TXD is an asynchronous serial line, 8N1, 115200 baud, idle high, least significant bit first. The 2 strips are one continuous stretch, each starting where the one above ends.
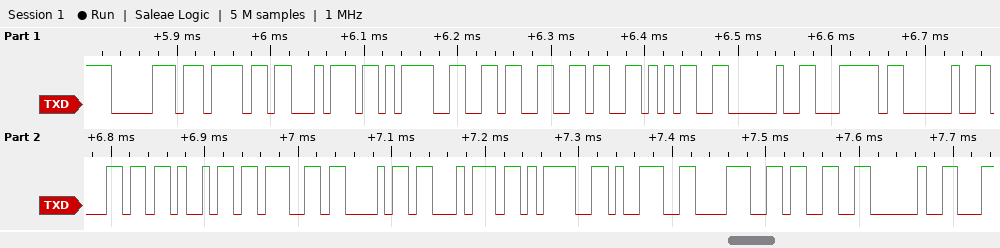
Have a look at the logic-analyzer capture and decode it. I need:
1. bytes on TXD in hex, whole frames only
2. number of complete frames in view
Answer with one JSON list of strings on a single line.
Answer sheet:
["0x70 0x6F 0x74 0x3D 0x36 0x36 0x35 0x20 0x7C 0x20 0x6C 0x69 0x67 0x68 0x74 0x3D 0x39 0x38 0x33 0x20", "20"]
